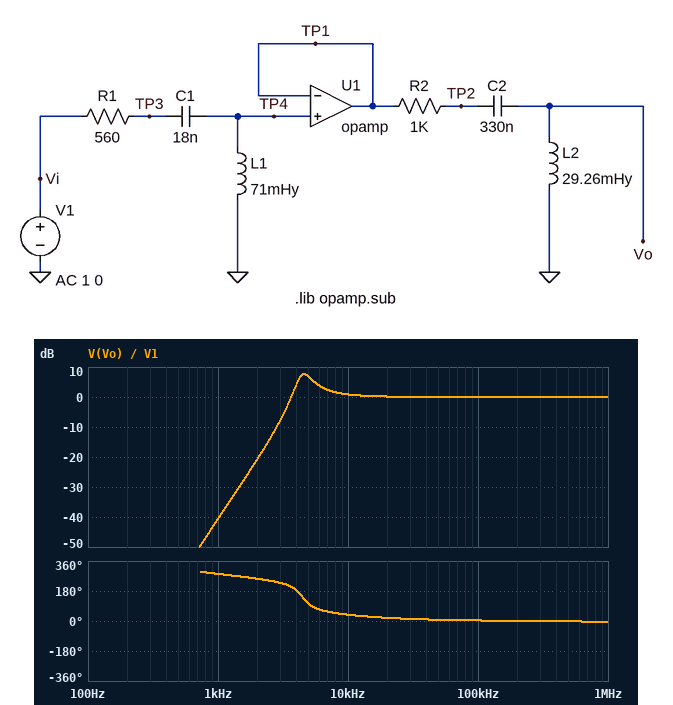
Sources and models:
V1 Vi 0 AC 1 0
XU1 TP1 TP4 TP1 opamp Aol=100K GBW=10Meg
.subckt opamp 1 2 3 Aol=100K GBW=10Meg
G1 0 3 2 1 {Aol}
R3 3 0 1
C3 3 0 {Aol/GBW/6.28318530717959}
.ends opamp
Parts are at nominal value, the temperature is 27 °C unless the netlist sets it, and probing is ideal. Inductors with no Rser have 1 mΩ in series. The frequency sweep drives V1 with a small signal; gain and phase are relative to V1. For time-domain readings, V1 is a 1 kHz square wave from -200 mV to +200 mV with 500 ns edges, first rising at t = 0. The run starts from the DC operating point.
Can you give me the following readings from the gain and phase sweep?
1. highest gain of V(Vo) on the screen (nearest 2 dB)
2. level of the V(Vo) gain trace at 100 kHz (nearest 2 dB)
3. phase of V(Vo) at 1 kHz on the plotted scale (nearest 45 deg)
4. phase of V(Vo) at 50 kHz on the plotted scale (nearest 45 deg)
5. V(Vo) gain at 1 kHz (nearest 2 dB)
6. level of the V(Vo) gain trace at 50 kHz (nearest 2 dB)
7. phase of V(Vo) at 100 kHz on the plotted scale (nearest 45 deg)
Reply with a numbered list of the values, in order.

1. 8 dB
2. 0 dB
3. 270 deg
4. 0 deg
5. -40 dB
6. 0 dB
7. 0 deg
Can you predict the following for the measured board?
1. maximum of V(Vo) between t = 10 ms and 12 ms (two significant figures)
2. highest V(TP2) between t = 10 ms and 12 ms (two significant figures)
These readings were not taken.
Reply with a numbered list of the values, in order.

1. 420 mV
2. 420 mV
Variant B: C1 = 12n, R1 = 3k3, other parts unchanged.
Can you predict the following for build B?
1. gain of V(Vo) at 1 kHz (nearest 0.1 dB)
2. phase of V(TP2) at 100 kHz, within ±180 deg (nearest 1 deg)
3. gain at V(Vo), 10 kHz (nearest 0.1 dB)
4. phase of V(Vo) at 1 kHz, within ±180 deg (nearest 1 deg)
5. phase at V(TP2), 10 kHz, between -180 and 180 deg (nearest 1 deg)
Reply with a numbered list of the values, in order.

1. -44.5 dB
2. 7 deg
3. -1.1 dB
4. -88 deg
5. 76 deg
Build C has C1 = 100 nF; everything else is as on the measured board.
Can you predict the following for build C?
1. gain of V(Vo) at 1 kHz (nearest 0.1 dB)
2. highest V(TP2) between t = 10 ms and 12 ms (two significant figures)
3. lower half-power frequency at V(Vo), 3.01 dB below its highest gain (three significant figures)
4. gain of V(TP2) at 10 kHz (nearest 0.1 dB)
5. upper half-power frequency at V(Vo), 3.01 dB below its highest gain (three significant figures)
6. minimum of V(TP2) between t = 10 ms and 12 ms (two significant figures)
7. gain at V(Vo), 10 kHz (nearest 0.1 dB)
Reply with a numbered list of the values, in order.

1. -24.2 dB
2. 410 mV
3. 3.16 kHz
4. -0.9 dB
5. 10.0 MHz
6. -410 mV
7. -0.7 dB
